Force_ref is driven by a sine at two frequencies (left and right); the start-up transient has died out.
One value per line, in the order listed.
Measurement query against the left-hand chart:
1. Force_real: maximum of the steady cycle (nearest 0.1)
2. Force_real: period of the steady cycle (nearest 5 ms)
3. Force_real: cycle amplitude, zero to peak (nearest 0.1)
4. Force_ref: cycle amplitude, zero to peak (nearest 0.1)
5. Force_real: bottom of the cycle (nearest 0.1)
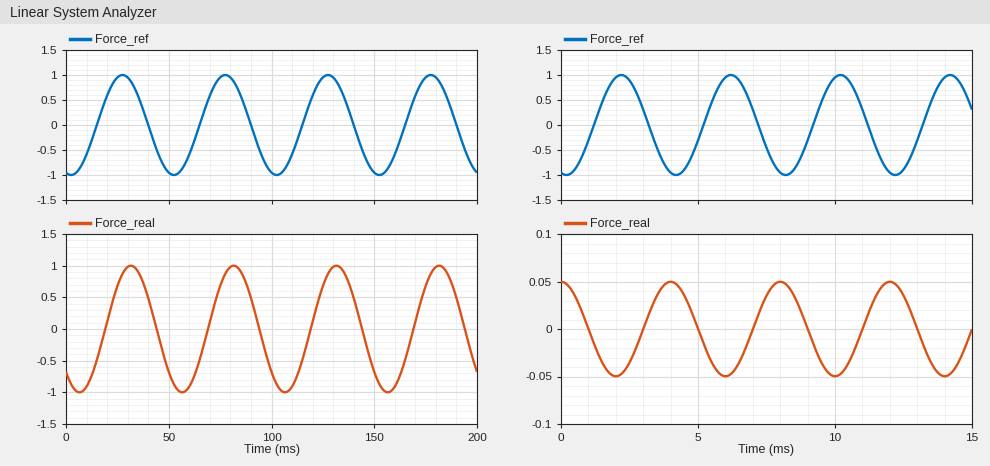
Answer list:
1.0
50 ms
1.0
1.0
-1.0
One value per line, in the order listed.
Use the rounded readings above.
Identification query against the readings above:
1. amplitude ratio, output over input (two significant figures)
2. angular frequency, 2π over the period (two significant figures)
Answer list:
1.0
0.13 rad/ms
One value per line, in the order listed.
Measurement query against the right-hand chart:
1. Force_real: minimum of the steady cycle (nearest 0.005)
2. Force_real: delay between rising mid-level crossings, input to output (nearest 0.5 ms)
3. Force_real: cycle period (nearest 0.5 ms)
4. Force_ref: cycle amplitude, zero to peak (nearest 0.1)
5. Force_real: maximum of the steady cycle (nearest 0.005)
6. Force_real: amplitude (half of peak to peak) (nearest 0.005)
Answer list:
-0.050
2.0 ms
4.0 ms
1.0
0.050
0.050
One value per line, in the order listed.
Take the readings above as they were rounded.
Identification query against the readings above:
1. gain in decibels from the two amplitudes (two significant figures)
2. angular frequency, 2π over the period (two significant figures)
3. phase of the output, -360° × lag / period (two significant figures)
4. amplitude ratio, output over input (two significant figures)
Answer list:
-26 dB
1.6 rad/ms
-180°
0.050
